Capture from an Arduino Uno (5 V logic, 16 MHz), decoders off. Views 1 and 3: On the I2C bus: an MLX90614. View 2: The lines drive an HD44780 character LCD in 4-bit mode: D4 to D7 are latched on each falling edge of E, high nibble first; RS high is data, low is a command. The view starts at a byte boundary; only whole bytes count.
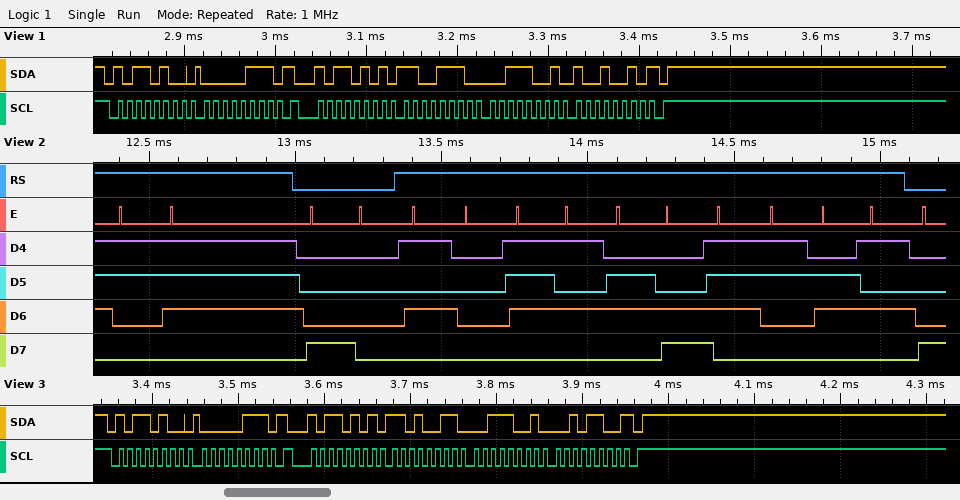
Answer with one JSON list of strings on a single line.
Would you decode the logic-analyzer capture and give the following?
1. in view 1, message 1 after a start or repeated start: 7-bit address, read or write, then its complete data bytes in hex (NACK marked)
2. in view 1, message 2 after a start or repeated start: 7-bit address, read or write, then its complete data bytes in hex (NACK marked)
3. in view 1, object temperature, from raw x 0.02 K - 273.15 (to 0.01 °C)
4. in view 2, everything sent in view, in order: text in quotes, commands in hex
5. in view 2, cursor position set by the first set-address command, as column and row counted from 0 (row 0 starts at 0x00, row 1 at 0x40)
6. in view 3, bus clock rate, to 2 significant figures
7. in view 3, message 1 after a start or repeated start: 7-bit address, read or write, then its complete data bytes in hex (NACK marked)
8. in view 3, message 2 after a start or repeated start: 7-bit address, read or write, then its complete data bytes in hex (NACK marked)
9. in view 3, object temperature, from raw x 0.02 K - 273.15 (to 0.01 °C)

["0x5A write: 07", "0x5A read: CE 39 92 NACK", "22.81 °C", "\"7\" 0x80 \"Pulse\"", "column 0, row 0", "100 kHz", "0x5A write: 07", "0x5A read: D3 39 2C NACK", "22.91 °C"]
